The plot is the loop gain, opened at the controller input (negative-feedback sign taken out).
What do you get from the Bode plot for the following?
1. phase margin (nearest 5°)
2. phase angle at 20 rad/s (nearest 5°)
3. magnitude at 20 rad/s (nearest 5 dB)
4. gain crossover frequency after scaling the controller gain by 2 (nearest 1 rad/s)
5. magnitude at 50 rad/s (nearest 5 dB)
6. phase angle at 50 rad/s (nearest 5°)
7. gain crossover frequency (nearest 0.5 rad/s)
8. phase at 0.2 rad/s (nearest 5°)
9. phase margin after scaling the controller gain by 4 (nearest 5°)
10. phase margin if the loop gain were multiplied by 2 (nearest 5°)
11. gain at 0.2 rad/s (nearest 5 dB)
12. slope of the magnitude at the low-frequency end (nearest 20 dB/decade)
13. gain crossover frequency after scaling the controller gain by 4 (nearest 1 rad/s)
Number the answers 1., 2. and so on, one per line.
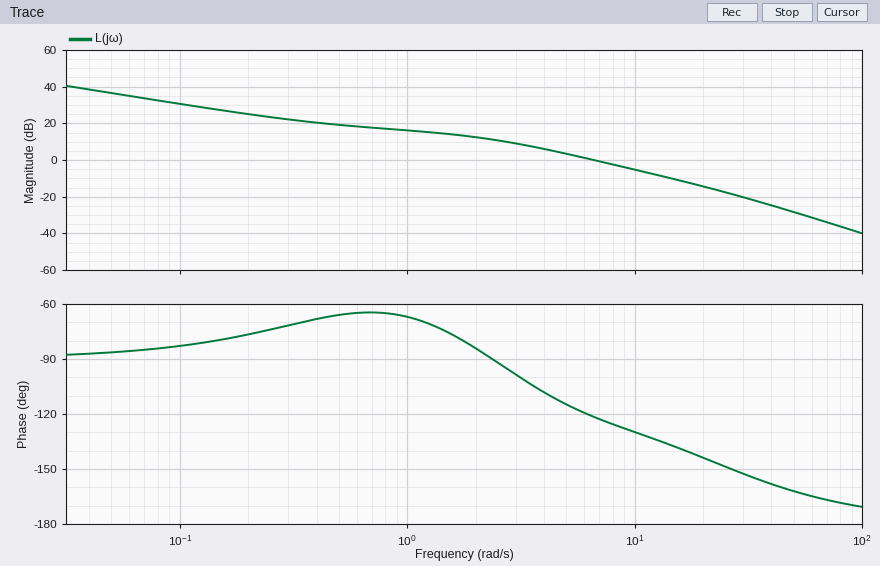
1. 60°
2. -145°
3. -15 dB
4. 11 rad/s
5. -30 dB
6. -160°
7. 6.5 rad/s
8. -75°
9. 40°
10. 50°
11. 25 dB
12. -20 dB/decade
13. 17 rad/s
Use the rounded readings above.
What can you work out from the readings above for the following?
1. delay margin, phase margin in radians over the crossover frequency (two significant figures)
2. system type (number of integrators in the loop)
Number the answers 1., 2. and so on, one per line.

1. 0.16 s
2. 1
